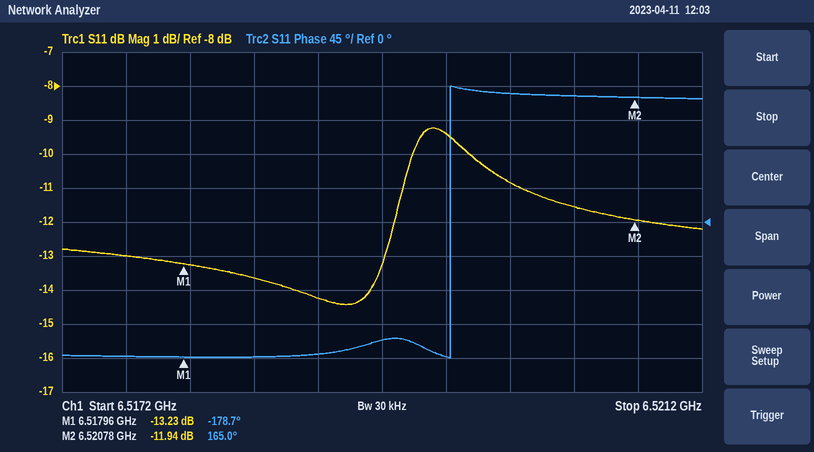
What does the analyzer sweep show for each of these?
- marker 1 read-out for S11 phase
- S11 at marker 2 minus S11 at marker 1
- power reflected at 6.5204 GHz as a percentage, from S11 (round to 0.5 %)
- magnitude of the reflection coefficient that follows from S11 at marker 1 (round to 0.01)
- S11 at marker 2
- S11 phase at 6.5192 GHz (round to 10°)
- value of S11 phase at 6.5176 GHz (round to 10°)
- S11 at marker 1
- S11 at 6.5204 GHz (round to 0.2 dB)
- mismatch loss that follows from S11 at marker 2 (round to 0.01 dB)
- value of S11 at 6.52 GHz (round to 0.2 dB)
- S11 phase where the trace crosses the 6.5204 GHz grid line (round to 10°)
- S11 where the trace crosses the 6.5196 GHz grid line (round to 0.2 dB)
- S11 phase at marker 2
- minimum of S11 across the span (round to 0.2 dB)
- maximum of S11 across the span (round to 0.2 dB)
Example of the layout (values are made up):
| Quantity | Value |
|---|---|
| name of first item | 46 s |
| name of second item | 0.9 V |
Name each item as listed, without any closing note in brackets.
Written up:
| Quantity | Value |
|---|---|
| marker 1 read-out for S11 phase | -178.7° |
| S11 at marker 2 minus S11 at marker 1 | 1.29 dB |
| power reflected at 6.5204 GHz as a percentage, from S11 | 7.0 % |
| magnitude of the reflection coefficient that follows from S11 at marker 1 | 0.22 |
| S11 at marker 2 | -11.94 dB |
| S11 phase at 6.5192 GHz | -160° |
| value of S11 phase at 6.5176 GHz | -180° |
| S11 at marker 1 | -13.23 dB |
| S11 at 6.5204 GHz | -11.6 dB |
| mismatch loss that follows from S11 at marker 2 | 0.29 dB |
| value of S11 at 6.52 GHz | -10.8 dB |
| S11 phase where the trace crosses the 6.5204 GHz grid line | 170° |
| S11 where the trace crosses the 6.5196 GHz grid line | -9.4 dB |
| S11 phase at marker 2 | 165.0° |
| minimum of S11 across the span | -14.4 dB |
| maximum of S11 across the span | -9.2 dB |
